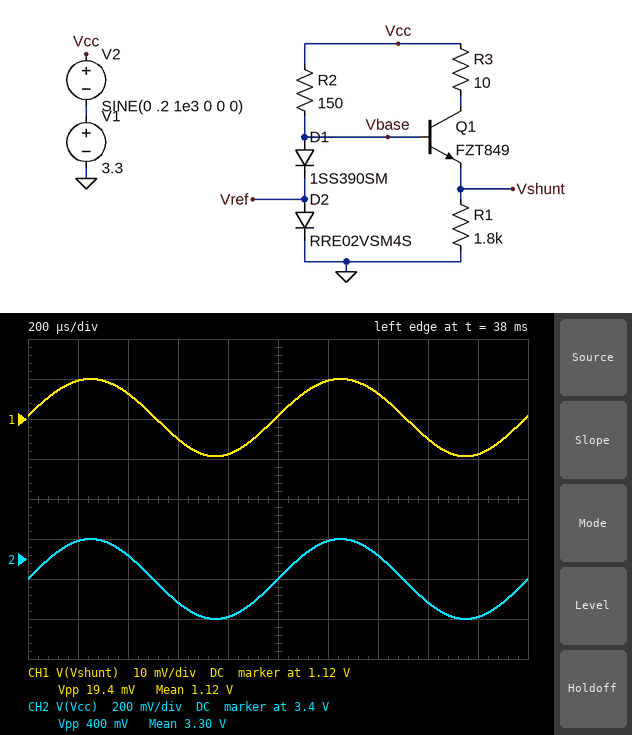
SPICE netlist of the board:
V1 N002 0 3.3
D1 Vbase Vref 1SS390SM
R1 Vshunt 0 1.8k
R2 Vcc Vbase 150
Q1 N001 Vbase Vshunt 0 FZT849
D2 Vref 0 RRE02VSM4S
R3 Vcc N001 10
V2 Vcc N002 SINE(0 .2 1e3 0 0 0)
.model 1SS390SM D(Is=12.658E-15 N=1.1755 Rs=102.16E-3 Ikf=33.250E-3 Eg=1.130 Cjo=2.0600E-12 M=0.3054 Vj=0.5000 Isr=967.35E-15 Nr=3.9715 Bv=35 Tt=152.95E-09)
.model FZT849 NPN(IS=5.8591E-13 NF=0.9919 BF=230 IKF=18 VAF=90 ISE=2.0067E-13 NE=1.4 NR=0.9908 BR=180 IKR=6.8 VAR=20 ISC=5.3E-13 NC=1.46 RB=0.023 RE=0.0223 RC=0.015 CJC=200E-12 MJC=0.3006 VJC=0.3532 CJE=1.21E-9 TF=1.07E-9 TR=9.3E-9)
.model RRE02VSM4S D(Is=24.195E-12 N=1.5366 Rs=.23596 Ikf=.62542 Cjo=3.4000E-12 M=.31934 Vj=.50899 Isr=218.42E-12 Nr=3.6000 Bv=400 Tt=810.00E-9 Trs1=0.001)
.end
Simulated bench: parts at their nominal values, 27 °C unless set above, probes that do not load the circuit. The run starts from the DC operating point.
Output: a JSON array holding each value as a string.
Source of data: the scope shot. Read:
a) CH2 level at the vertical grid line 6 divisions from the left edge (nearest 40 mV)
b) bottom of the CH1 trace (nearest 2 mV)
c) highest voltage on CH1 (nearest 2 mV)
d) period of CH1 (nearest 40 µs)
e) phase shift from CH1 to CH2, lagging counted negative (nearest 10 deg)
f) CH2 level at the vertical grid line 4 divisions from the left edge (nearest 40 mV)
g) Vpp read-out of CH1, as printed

["3.48 V", "1.110 V", "1.130 V", "1.00 ms", "0 deg", "3.12 V", "19.4 mV"]
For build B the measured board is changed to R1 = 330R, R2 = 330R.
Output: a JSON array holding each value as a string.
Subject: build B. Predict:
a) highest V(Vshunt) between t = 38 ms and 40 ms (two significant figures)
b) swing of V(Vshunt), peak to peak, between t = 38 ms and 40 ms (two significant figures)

["1.0 V", "18 mV"]
